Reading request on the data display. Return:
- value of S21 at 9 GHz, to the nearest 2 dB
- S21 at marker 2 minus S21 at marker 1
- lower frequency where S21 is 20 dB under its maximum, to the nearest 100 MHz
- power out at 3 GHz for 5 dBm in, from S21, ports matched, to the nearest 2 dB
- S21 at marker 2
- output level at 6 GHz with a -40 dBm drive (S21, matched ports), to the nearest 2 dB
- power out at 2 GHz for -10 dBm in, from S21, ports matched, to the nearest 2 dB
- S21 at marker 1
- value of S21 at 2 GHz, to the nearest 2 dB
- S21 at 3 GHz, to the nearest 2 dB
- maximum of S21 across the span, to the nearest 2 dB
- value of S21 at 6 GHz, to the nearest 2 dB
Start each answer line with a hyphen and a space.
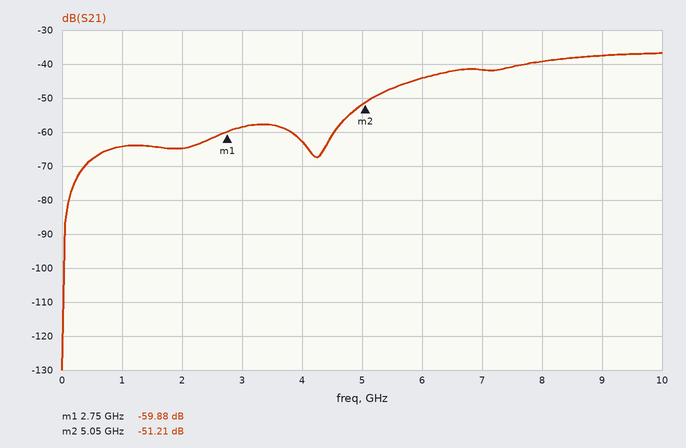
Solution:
- -38 dB
- 8.67 dB
- 4.7 GHz
- -54 dBm
- -51.21 dB
- -84 dBm
- -74 dBm
- -59.88 dB
- -64 dB
- -58 dB
- -36 dB
- -44 dB
